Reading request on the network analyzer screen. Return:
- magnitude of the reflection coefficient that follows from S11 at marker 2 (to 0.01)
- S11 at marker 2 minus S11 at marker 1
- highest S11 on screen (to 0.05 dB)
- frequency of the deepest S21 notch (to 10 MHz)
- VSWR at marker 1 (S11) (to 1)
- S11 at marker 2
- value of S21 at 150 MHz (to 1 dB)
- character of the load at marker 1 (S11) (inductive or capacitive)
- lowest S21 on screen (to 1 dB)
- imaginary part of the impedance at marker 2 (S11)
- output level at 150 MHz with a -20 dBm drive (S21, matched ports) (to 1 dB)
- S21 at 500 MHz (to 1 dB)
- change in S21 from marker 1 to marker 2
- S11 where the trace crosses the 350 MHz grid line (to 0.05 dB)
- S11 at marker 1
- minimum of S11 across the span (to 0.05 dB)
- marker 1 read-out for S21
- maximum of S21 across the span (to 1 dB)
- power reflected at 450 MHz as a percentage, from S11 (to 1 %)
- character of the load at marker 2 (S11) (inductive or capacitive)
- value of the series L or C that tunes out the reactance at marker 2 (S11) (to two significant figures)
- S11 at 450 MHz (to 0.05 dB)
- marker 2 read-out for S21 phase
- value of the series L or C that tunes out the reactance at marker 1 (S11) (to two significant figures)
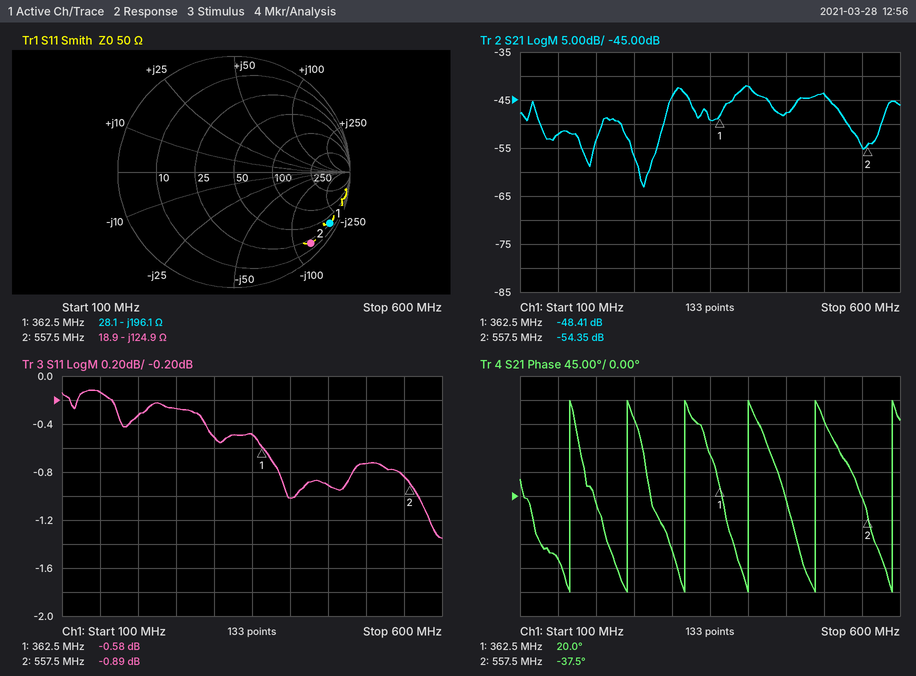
0.90
-0.31 dB
-0.10 dB
260 MHz
30
-0.89 dB
-52 dB
capacitive
-63 dB
-124.9 Ω
-72 dBm
-44 dB
-5.94 dB
-0.50 dB
-0.58 dB
-1.35 dB
-48.41 dB
-42 dB
81 %
capacitive
36 nH
-0.90 dB
-37.5°
86 nH
